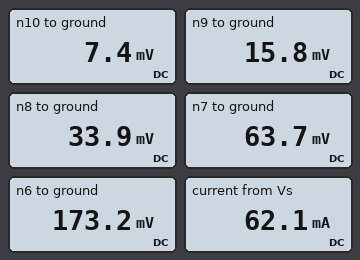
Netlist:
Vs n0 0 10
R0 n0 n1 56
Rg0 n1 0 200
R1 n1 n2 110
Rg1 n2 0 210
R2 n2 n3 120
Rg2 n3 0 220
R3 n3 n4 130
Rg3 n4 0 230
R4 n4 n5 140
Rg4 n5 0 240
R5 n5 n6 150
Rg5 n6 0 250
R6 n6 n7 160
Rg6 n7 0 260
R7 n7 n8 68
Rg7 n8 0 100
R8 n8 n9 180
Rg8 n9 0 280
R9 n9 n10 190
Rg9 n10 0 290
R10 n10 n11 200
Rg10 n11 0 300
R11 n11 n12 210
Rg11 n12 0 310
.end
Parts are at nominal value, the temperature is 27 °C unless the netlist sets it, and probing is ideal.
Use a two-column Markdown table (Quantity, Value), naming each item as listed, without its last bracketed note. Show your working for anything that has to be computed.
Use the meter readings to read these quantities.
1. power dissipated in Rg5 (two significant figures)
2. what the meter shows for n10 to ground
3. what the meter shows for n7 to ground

| Quantity | Value |
|---|---|
| power dissipated in Rg5 | (173.2 mV)^2 / 250 Ω = 120 µW |
| what the meter shows for n10 to ground | 7.4 mV |
| what the meter shows for n7 to ground | 63.7 mV |
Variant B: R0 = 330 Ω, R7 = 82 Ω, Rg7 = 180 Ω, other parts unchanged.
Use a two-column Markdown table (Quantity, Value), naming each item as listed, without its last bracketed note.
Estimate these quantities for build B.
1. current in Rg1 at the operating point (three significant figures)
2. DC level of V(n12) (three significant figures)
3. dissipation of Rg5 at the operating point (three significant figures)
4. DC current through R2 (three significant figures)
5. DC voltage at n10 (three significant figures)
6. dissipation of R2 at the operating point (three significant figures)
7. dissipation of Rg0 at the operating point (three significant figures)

| Quantity | Value |
|---|---|
| current in Rg1 at the operating point | 5.79 mA |
| DC level of V(n12) | 1.01 mV |
| dissipation of Rg5 at the operating point | 17.3 µW |
| DC current through R2 | 5.11 mA |
| DC voltage at n10 | 3.48 mV |
| dissipation of R2 at the operating point | 3.14 mW |
| dissipation of Rg0 at the operating point | 29.2 mW |
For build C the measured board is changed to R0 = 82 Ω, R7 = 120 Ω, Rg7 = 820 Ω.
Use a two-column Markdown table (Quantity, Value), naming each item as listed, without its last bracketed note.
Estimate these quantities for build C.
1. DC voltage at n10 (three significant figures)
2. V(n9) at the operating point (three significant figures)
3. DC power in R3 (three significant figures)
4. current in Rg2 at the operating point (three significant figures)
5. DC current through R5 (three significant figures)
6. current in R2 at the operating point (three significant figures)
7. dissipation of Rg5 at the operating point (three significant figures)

| Quantity | Value |
|---|---|
| DC voltage at n10 | 11.2 mV |
| V(n9) at the operating point | 23.9 mV |
| DC power in R3 | 3.95 mW |
| current in Rg2 at the operating point | 6.37 mA |
| DC current through R5 | 1.15 mA |
| current in R2 at the operating point | 11.9 mA |
| dissipation of Rg5 at the operating point | 101 µW |
